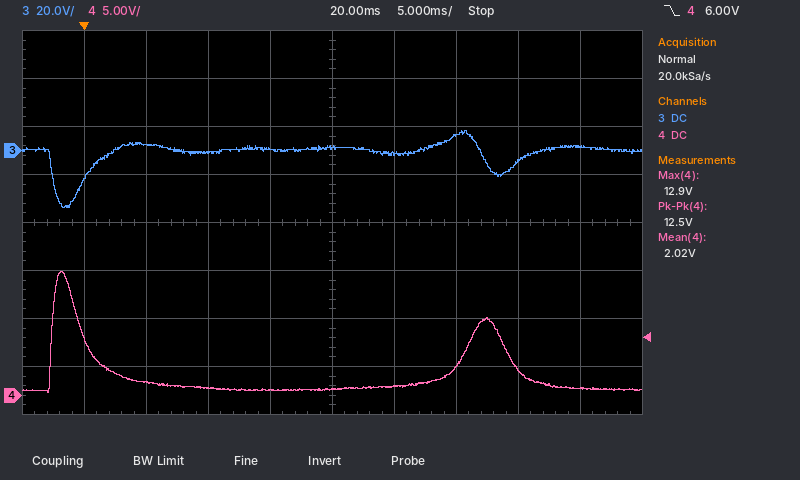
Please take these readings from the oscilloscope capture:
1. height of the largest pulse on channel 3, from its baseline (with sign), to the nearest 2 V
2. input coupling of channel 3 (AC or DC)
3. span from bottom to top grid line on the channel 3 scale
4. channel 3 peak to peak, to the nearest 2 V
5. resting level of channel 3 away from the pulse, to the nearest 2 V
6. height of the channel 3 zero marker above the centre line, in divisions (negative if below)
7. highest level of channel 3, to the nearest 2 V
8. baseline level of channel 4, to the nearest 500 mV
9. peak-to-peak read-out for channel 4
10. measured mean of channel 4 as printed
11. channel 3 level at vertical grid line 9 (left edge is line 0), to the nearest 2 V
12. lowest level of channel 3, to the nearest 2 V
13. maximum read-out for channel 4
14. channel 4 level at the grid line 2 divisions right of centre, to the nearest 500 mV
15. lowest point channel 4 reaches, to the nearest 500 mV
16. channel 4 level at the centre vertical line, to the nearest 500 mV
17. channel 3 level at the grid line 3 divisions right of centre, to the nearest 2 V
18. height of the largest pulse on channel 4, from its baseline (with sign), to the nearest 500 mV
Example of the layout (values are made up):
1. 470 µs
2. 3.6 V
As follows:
1. -24 V
2. DC
3. 160 V
4. 32 V
5. 0 V
6. +1.5 div
7. 8 V
8. 500 mV
9. 12.5 V
10. 2.02 V
11. 2 V
12. -24 V
13. 12.9 V
14. 3.0 V
15. 500 mV
16. 500 mV
17. -4 V
18. +12.0 V
